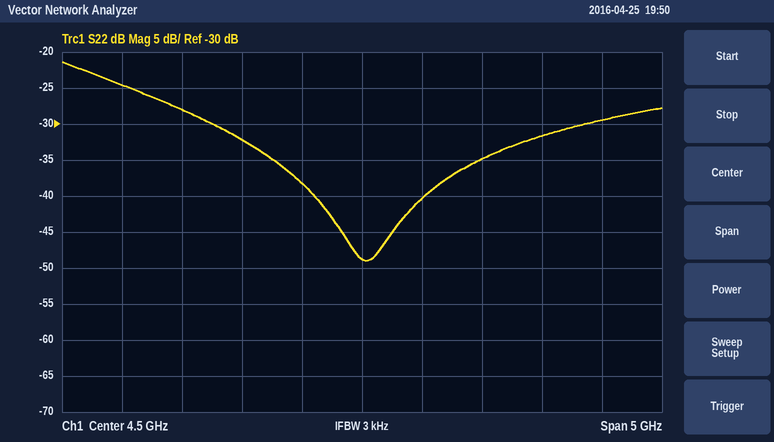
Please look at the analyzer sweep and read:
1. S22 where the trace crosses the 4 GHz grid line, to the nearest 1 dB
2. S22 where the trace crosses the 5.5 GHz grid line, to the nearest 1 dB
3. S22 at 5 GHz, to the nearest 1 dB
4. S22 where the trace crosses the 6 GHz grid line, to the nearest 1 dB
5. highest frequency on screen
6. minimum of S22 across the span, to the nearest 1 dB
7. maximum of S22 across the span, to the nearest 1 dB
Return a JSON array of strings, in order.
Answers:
["-38 dB", "-35 dB", "-40 dB", "-32 dB", "7 GHz", "-49 dB", "-21 dB"]
